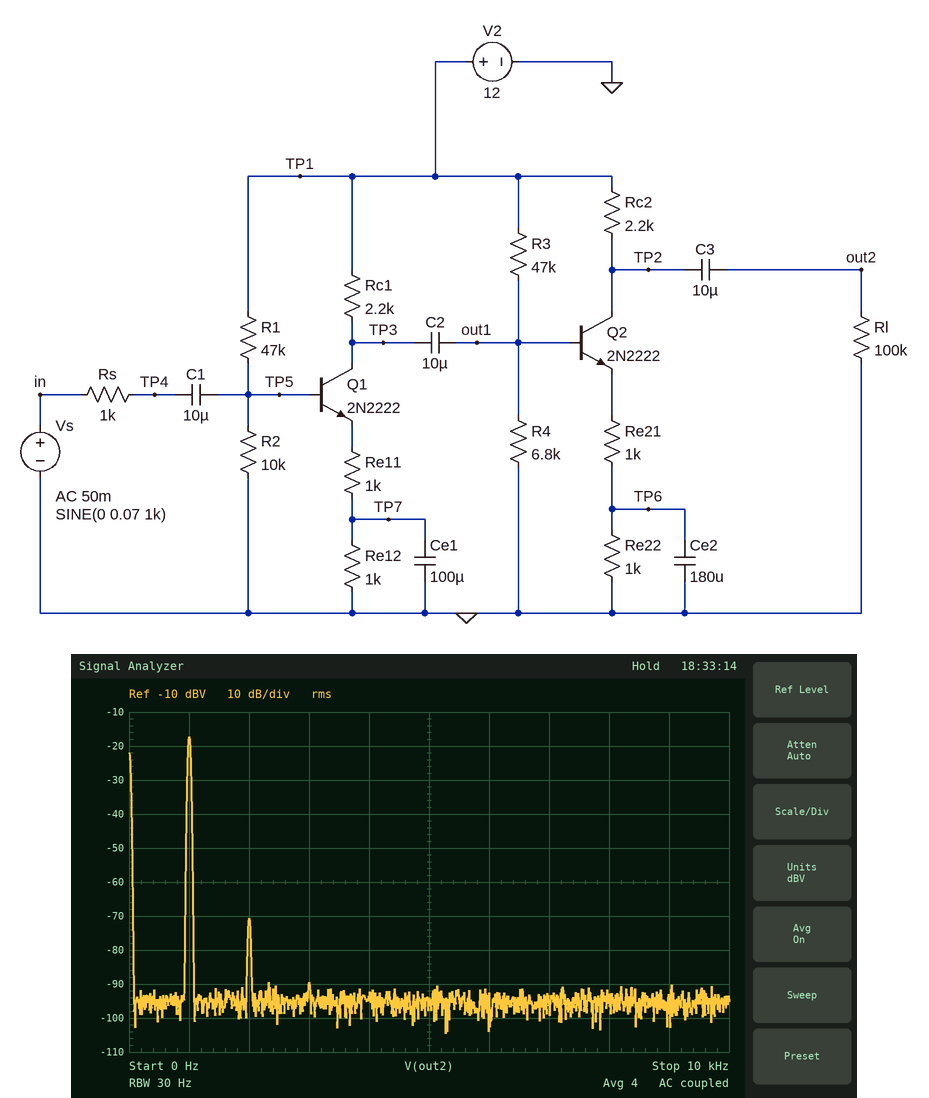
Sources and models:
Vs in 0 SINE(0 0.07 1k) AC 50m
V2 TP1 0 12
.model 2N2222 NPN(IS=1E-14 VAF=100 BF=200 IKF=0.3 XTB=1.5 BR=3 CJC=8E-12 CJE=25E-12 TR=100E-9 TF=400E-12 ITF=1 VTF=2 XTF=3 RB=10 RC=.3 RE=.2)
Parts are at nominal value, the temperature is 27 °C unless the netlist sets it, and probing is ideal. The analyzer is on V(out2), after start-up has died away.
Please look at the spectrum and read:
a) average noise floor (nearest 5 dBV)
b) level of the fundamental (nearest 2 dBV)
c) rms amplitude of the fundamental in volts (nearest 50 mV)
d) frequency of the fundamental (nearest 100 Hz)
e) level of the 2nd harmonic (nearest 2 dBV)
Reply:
-95 dBV
-18 dBV
150 mV
1.0 kHz
-70 dBV
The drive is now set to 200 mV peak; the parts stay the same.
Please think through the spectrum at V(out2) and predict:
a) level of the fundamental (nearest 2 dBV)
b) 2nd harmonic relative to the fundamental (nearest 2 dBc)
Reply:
-8 dBV
-42 dBc
